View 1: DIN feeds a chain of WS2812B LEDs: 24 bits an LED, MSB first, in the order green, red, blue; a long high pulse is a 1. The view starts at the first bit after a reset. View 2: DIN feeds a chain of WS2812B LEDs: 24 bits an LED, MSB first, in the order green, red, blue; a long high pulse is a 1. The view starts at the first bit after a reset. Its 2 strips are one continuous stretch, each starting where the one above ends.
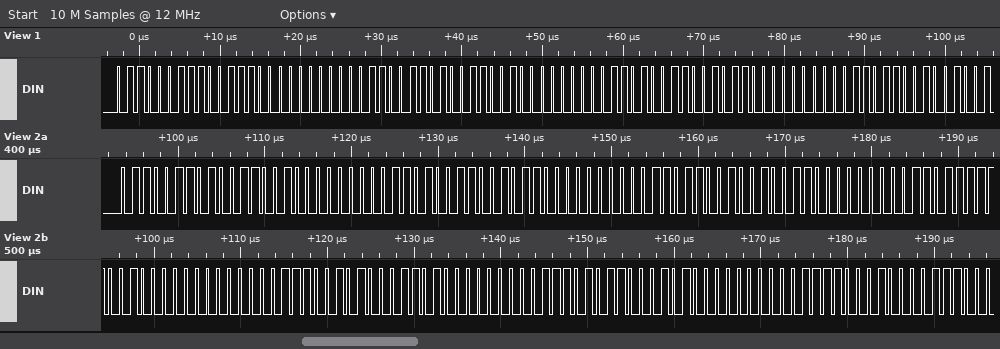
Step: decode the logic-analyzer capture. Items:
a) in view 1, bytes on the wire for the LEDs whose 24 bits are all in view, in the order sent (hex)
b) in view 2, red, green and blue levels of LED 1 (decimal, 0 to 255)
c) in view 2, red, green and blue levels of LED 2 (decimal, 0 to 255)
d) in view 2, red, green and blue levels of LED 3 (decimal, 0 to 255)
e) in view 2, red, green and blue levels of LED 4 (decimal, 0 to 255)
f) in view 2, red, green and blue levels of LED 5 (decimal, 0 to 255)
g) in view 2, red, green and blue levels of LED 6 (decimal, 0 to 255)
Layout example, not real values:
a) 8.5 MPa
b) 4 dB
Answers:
a) 63 9C 00 66 99 00 69 96 00
b) 153, 102, 0
c) 150, 105, 0
d) 147, 108, 0
e) 144, 111, 0
f) 141, 114, 0
g) 138, 117, 0
